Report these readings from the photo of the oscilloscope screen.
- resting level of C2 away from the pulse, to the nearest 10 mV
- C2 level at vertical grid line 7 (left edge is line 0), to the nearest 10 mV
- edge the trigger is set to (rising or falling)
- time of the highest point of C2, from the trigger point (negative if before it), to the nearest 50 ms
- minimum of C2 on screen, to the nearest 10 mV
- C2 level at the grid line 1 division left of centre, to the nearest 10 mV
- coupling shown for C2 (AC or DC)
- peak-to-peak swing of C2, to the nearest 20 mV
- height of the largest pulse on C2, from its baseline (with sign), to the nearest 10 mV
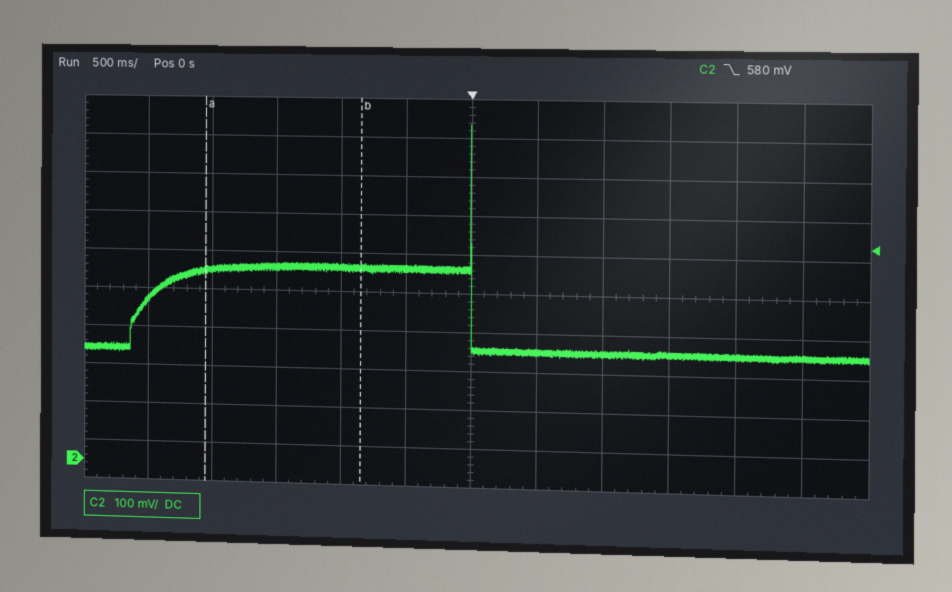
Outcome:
300 mV
300 mV
falling
0 ms
290 mV
510 mV
DC
600 mV
+580 mV
